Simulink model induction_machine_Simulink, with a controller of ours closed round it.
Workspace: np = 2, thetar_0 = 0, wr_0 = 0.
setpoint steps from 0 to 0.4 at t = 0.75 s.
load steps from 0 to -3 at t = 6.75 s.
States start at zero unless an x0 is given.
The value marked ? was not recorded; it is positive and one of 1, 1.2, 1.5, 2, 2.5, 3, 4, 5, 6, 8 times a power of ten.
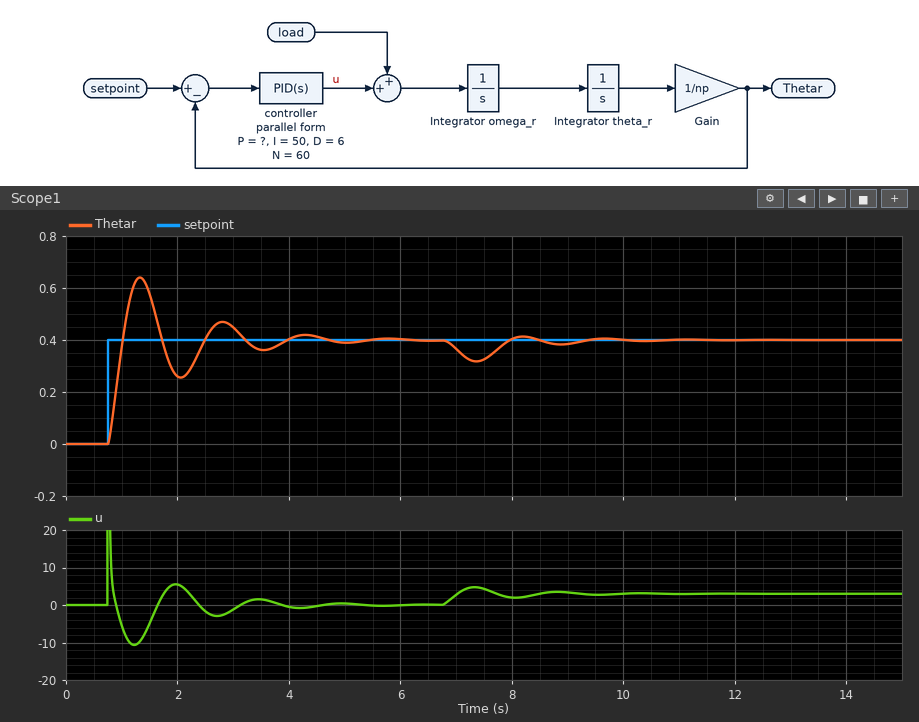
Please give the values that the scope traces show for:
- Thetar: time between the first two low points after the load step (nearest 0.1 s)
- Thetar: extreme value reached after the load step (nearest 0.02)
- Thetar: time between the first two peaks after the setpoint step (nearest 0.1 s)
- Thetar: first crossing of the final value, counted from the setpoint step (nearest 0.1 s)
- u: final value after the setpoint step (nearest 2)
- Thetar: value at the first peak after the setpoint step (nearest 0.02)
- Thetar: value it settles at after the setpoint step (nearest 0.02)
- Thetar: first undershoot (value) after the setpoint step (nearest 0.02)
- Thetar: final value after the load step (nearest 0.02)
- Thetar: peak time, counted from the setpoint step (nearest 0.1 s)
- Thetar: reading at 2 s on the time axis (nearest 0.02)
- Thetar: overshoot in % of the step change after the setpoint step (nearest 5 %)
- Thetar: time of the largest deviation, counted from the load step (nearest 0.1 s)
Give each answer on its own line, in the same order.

1.5 s
0.32
1.5 s
0.3 s
0
0.64
0.40
0.26
0.40
0.6 s
0.26
60 %
0.6 s
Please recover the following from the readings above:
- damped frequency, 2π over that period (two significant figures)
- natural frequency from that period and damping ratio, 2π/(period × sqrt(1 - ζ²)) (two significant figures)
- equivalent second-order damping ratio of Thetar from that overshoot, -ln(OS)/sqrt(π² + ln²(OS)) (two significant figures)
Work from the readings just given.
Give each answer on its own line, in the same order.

4.2 rad/s
4.2 rad/s
0.16
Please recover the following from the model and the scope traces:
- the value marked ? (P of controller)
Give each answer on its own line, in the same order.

40
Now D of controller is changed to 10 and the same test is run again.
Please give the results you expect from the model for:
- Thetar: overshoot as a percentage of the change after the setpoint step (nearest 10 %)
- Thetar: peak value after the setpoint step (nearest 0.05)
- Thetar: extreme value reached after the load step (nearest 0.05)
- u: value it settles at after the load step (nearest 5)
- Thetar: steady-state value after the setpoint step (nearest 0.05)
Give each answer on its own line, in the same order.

40 %
0.55
0.35
5
0.40
